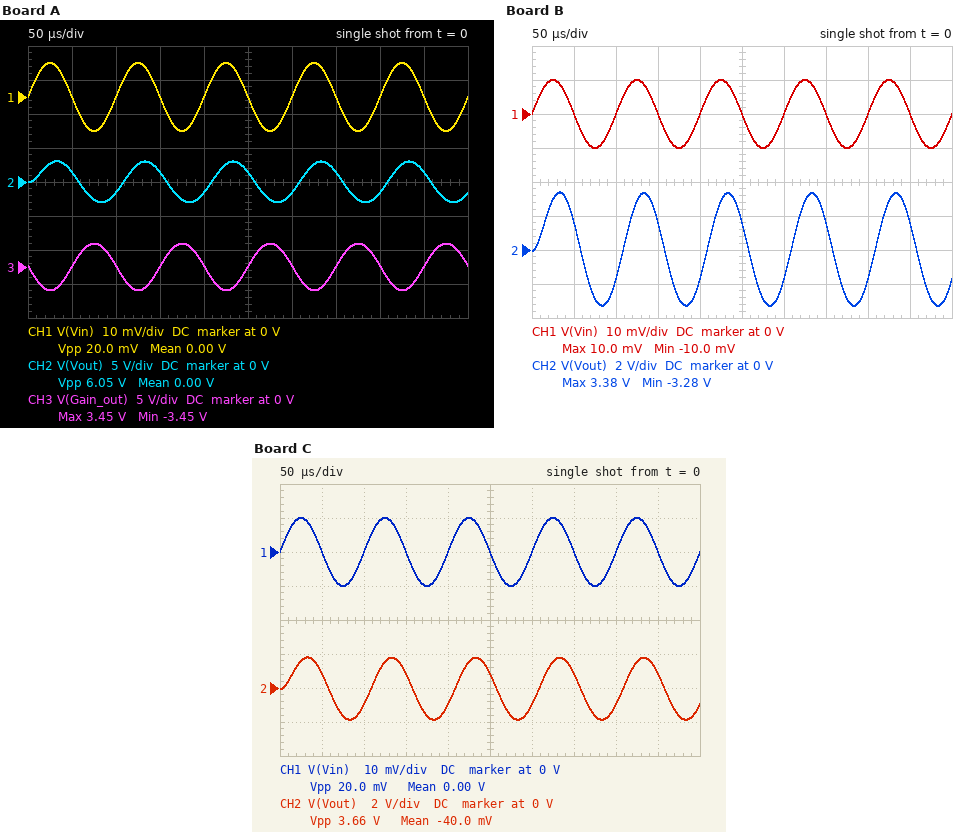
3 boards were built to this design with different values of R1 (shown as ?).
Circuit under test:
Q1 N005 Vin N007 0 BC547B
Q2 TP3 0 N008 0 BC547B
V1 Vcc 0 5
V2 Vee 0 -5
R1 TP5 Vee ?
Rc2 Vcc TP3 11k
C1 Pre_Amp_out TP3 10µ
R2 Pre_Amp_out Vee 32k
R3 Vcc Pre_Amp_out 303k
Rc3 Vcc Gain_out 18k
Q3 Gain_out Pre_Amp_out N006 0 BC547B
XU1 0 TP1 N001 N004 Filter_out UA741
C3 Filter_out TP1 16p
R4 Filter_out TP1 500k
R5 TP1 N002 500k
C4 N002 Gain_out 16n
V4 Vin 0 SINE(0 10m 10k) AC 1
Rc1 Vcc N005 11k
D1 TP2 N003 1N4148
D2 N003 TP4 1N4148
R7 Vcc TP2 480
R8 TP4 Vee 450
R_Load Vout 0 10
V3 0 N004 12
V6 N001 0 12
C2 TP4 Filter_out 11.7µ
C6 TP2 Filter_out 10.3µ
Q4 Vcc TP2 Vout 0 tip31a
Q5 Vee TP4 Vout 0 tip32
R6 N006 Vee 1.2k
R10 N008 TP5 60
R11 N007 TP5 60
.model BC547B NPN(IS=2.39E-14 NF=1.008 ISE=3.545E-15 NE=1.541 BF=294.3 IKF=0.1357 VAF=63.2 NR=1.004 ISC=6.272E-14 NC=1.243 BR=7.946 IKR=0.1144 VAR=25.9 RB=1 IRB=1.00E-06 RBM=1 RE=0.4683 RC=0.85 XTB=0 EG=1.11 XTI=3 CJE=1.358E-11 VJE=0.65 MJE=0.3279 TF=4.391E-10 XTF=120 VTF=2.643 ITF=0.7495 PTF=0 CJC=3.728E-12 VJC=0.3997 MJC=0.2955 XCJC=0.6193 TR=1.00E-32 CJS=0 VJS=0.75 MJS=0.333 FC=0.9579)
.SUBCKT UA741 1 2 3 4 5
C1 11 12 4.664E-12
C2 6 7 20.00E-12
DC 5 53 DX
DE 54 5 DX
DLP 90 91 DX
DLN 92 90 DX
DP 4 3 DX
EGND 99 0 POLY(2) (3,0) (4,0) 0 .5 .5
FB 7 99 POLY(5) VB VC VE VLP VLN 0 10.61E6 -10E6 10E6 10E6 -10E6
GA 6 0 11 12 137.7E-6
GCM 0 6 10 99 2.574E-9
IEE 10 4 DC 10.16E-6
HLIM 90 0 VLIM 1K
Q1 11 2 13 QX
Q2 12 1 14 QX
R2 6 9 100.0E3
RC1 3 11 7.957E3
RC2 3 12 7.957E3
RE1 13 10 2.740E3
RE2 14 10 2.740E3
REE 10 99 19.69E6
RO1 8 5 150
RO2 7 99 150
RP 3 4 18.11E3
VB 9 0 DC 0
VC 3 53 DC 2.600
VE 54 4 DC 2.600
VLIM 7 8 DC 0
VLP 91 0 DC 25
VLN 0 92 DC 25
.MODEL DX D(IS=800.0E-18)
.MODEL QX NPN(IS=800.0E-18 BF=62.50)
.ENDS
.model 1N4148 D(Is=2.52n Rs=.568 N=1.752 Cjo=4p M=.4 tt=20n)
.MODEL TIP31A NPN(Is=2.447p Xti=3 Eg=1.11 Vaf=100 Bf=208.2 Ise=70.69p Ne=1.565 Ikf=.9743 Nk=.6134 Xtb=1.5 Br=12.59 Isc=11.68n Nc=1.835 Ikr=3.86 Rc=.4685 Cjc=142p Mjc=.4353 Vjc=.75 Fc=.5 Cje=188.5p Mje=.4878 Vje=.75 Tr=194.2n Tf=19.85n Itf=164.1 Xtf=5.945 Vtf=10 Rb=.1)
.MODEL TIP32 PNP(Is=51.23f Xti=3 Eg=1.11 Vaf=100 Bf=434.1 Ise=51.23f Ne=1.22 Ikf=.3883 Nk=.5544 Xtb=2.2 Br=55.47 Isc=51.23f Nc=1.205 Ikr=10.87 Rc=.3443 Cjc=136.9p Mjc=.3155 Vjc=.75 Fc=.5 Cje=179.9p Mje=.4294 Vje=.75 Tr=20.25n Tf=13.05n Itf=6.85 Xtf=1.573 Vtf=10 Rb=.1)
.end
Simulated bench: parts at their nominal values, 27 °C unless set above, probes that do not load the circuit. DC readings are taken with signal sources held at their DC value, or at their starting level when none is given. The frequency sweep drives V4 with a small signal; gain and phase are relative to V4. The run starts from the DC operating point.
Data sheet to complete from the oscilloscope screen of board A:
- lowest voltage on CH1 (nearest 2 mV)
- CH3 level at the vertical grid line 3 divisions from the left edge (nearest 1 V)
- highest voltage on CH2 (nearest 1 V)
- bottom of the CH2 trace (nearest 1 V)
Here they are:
-10 mV
0 V
3 V
-3 V
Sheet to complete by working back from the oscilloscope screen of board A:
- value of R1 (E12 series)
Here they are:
6.8 kΩ
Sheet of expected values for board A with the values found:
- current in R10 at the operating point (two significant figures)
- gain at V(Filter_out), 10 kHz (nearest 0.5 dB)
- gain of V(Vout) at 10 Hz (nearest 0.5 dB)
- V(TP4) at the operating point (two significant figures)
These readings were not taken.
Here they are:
320 µA
50.0 dB
32.0 dB
-800 mV
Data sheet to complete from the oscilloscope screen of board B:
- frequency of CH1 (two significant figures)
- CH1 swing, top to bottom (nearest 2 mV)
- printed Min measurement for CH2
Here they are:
10 kHz
20 mV
-3.28 V
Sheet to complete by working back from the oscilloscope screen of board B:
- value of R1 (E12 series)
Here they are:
5.6 kΩ
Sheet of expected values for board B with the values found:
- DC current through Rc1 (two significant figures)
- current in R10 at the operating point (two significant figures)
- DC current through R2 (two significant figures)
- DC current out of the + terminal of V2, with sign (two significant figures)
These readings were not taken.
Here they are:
390 µA
390 µA
29 µA
-110 mA
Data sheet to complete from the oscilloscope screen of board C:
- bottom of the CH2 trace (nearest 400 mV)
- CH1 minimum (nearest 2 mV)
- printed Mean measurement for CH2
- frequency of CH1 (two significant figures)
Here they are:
-2.0 V
-10 mV
-40.0 mV
10 kHz
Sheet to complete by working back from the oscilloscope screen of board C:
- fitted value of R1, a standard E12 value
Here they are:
15 kΩ
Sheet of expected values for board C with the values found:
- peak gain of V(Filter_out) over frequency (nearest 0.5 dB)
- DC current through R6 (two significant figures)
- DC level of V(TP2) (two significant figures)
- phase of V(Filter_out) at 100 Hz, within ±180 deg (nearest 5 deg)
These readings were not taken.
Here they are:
46.5 dB
270 µA
570 mV
10 deg
